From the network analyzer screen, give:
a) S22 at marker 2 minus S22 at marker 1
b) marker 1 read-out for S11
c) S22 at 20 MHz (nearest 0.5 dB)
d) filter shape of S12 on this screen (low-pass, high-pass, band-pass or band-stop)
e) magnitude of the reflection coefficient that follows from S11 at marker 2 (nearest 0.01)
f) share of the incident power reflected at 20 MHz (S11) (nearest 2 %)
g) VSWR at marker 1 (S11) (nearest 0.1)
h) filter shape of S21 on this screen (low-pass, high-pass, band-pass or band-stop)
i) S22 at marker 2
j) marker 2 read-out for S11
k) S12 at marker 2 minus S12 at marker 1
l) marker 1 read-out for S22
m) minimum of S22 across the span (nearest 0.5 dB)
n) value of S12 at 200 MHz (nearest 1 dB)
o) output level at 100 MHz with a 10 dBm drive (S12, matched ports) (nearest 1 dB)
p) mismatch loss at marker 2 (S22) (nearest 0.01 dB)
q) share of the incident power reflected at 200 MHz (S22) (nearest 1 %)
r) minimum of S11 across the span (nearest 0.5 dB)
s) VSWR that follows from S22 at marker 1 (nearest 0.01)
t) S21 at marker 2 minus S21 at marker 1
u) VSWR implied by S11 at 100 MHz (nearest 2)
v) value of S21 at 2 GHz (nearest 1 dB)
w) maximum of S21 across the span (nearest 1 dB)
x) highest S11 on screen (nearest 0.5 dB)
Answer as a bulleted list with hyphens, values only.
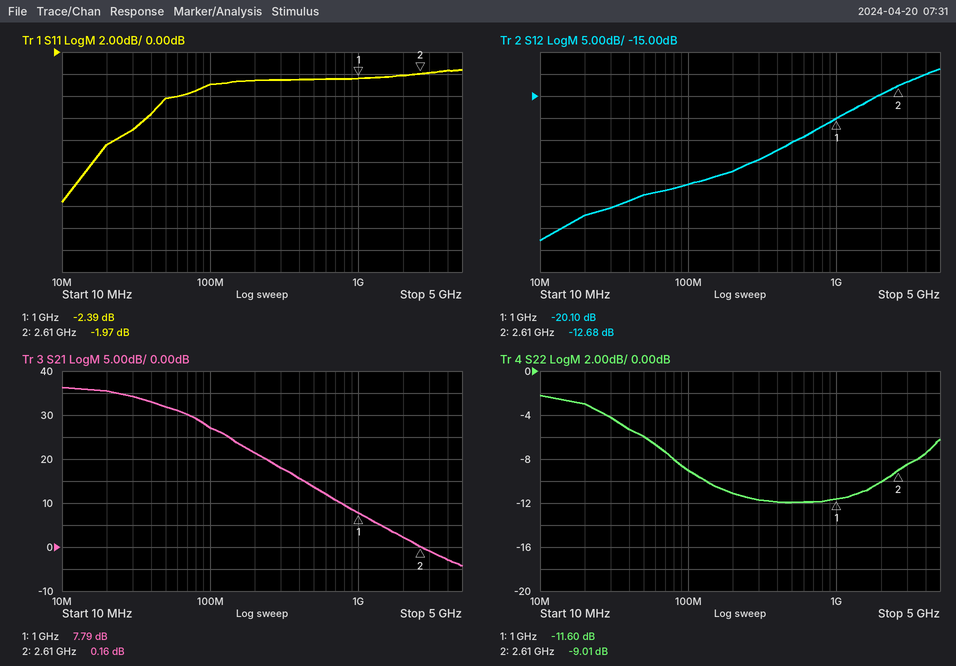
- 2.59 dB
- -2.39 dB
- -3.0 dB
- high-pass
- 0.80
- 14 %
- 7.3
- low-pass
- -9.01 dB
- -1.97 dB
- 7.42 dB
- -11.60 dB
- -12.0 dB
- -32 dB
- -25 dBm
- 0.58 dB
- 8 %
- -13.5 dB
- 1.71
- -7.63 dB
- 6
- 2 dB
- 36 dB
- -1.5 dB
